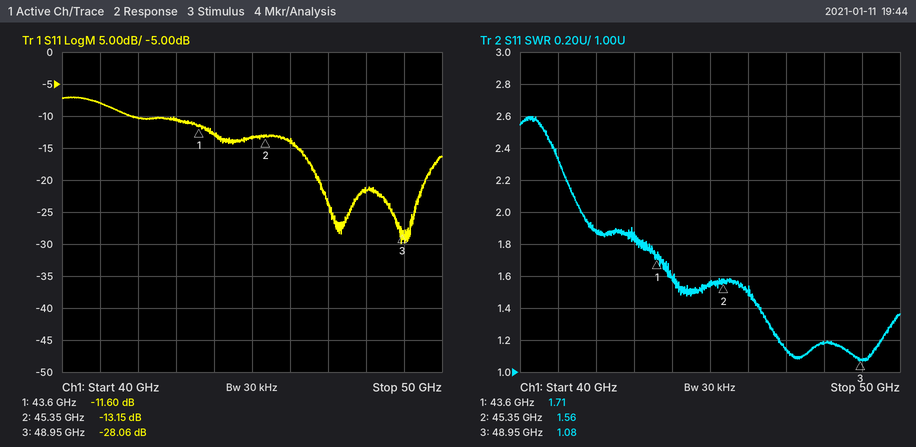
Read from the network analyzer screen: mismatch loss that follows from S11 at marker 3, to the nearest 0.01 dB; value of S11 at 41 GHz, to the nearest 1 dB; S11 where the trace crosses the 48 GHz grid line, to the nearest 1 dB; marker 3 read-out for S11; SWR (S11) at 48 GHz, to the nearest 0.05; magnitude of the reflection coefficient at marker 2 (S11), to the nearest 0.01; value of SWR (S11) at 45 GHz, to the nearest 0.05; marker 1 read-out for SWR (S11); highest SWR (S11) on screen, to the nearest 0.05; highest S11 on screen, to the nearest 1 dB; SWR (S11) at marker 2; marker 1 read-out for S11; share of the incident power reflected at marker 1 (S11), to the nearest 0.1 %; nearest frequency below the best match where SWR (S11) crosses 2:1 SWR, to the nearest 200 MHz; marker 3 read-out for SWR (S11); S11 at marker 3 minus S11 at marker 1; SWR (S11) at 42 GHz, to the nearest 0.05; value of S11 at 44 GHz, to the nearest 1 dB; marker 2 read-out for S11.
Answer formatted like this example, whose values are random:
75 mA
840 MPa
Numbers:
0.01 dB
-8 dB
-22 dB
-28.06 dB
1.20
0.22
1.55
1.71
2.60
-7 dB
1.56
-11.60 dB
6.9 %
41.6 GHz
1.08
-16.46 dB
1.90
-13 dB
-13.15 dB
